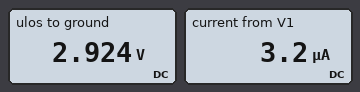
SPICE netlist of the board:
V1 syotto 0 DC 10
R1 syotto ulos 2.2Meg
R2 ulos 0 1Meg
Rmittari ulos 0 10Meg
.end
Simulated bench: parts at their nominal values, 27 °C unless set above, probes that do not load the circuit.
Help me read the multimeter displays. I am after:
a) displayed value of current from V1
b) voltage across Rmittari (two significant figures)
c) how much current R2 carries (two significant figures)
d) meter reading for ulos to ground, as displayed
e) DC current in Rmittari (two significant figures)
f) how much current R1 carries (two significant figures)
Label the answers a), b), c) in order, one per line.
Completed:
a) 3.2 µA
b) 2.9 V
c) 2.9 µA
d) 2.924 V
e) 290 nA
f) 3.2 µA
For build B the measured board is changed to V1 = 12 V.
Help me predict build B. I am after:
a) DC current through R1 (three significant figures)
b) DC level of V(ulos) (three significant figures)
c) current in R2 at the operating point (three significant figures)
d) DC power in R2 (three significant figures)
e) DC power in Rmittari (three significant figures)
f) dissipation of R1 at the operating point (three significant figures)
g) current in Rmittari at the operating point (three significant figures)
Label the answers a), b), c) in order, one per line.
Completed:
a) 3.86 µA
b) 3.51 V
c) 3.51 µA
d) 12.3 µW
e) 1.23 µW
f) 32.8 µW
g) 351 nA
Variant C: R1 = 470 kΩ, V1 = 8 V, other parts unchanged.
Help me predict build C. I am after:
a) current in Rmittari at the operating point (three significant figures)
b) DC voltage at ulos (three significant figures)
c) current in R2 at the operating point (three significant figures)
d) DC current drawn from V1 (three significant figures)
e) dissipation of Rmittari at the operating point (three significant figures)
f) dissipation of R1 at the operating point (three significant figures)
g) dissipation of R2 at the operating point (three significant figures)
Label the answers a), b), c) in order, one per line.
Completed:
a) 527 nA
b) 5.27 V
c) 5.27 µA
d) 5.80 µA
e) 2.78 µW
f) 15.8 µW
g) 27.8 µW
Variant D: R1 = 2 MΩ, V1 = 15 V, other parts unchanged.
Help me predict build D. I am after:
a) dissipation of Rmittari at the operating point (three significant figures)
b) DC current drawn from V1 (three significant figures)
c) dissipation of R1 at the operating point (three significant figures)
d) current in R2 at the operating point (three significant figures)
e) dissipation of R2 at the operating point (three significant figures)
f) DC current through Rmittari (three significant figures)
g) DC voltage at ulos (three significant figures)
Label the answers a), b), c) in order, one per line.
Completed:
a) 2.20 µW
b) 5.16 µA
c) 53.2 µW
d) 4.69 µA
e) 22.0 µW
f) 469 nA
g) 4.69 V
